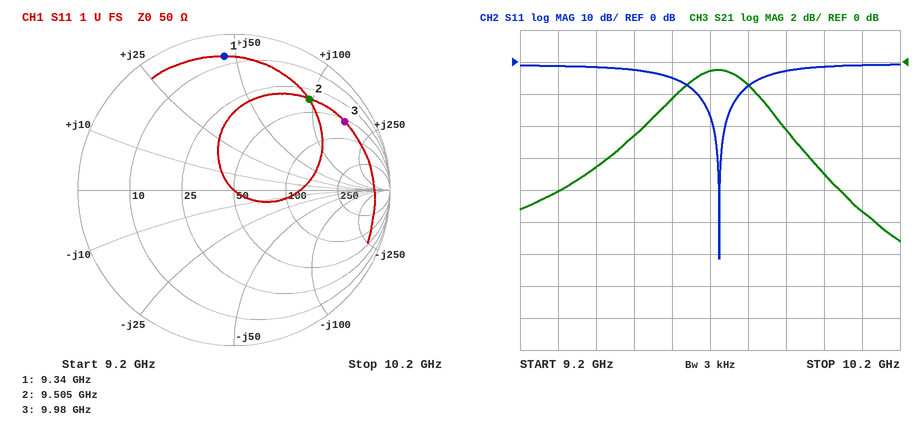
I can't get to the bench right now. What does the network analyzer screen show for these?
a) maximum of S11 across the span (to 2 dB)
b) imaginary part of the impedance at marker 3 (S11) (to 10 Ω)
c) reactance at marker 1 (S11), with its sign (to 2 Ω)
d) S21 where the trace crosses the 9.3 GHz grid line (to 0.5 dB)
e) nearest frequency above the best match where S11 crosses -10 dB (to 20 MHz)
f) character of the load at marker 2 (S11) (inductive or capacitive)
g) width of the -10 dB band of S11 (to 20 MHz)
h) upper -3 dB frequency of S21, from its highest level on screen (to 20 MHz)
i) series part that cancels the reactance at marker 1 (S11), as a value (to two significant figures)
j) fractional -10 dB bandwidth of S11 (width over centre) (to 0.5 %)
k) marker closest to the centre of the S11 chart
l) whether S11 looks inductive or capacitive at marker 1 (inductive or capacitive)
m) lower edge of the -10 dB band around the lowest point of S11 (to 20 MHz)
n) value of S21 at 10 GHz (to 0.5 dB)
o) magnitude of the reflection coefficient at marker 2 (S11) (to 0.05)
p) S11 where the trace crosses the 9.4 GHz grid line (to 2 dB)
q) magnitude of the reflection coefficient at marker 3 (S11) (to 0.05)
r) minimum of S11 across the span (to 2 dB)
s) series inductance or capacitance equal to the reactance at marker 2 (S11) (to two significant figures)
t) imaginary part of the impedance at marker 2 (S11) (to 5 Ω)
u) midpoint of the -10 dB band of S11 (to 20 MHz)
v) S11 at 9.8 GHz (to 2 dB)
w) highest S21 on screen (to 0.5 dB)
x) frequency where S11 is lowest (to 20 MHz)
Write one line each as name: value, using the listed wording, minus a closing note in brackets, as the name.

maximum of S11 across the span: 0 dB
imaginary part of the impedance at marker 3 (S11): +160 Ω
reactance at marker 1 (S11), with its sign: +46 Ω
S21 where the trace crosses the 9.3 GHz grid line: -8.0 dB
nearest frequency above the best match where S11 crosses -10 dB: 9.78 GHz
character of the load at marker 2 (S11): inductive
width of the -10 dB band of S11: 120 MHz
upper -3 dB frequency of S21, from its highest level on screen: 9.88 GHz
series part that cancels the reactance at marker 1 (S11), as a value: 370 fF
fractional -10 dB bandwidth of S11 (width over centre): 1.0 %
marker closest to the centre of the S11 chart: marker 2
whether S11 looks inductive or capacitive at marker 1: inductive
lower edge of the -10 dB band around the lowest point of S11: 9.66 GHz
value of S21 at 10 GHz: -7.0 dB
magnitude of the reflection coefficient at marker 2 (S11): 0.75
S11 where the trace crosses the 9.4 GHz grid line: -2 dB
magnitude of the reflection coefficient at marker 3 (S11): 0.85
minimum of S11 across the span: -62 dB
series inductance or capacitance equal to the reactance at marker 2 (S11): 1.6 nH
imaginary part of the impedance at marker 2 (S11): +95 Ω
midpoint of the -10 dB band of S11: 9.72 GHz
S11 at 9.8 GHz: -8 dB
highest S21 on screen: -0.5 dB
frequency where S11 is lowest: 9.72 GHz
